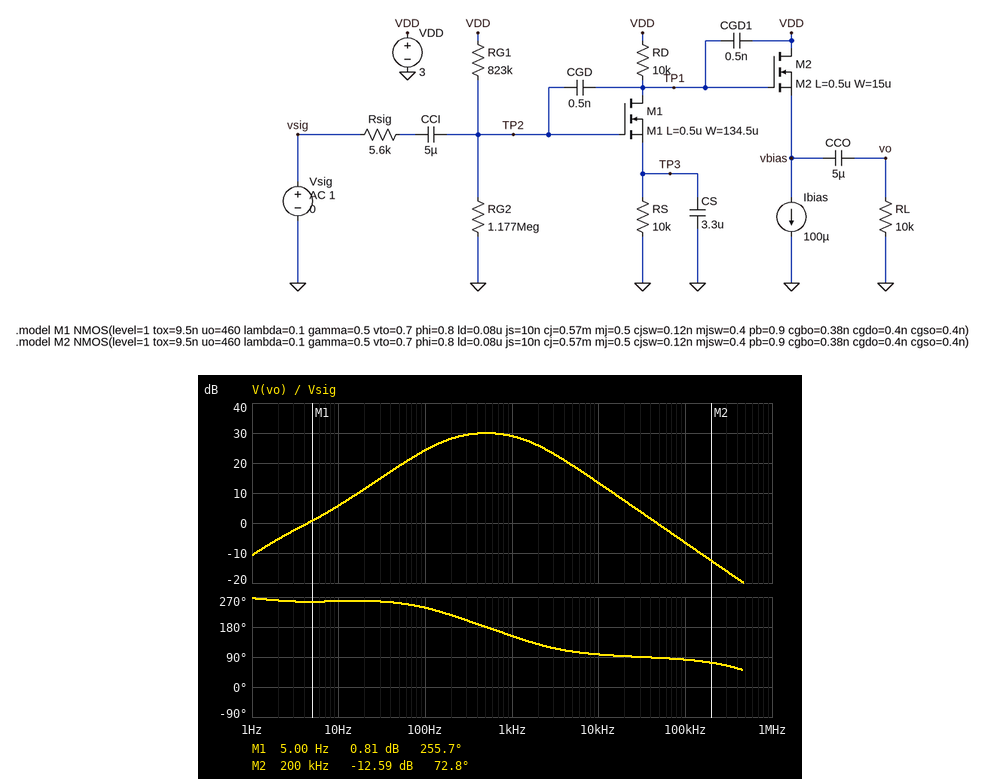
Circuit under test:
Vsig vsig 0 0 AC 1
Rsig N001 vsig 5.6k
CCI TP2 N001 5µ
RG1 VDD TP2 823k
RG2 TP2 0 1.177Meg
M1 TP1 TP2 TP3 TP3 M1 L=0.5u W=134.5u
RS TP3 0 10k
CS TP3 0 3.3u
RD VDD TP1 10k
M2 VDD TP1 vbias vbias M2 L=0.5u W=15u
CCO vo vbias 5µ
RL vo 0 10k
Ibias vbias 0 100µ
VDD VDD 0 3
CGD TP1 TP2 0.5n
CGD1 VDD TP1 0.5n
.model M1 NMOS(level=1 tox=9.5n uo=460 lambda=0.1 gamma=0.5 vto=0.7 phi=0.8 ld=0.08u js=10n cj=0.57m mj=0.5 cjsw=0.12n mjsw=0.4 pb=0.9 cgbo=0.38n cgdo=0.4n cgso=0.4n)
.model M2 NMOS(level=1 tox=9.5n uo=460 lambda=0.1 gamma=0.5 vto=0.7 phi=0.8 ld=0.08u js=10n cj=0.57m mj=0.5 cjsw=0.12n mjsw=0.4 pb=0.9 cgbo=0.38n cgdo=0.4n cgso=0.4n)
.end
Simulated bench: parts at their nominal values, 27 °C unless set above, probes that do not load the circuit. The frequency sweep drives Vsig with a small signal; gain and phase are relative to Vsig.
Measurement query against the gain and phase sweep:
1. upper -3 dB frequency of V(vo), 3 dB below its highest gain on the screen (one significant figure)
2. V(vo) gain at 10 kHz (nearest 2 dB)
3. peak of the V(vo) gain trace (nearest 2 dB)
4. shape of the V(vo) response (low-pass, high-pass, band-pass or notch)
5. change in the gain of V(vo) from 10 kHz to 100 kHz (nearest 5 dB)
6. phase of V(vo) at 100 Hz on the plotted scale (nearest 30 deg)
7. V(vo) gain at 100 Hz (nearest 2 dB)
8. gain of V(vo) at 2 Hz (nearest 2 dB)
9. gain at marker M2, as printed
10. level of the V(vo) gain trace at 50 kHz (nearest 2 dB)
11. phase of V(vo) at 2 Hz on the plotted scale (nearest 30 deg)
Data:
2 kHz
14 dB
30 dB
band-pass
-20 dB
240 deg
24 dB
-6 dB
-12.59 dB
0 dB
270 deg
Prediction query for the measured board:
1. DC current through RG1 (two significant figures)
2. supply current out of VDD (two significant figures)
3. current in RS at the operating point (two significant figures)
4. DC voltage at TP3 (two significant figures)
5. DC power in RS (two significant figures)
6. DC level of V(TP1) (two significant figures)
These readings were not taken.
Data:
1.5 µA
200 µA
100 µA
1.0 V
100 µW
2.0 V
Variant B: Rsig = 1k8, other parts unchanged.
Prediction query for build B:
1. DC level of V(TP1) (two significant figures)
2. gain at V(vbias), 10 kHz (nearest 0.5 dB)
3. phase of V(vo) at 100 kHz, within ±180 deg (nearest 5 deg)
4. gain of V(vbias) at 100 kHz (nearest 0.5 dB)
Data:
2.0 V
21.5 dB
85 deg
2.0 dB
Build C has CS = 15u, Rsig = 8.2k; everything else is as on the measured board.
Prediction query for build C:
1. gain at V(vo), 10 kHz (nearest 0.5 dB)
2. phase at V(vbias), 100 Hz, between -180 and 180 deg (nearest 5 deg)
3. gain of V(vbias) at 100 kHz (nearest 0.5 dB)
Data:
10.5 dB
-165 deg
-9.5 dB
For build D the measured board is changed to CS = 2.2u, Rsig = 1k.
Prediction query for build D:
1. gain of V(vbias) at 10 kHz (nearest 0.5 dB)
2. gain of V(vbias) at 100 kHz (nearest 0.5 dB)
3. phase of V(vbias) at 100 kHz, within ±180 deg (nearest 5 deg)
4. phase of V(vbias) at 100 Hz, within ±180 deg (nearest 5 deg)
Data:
24.5 dB
5.5 dB
85 deg
-115 deg
